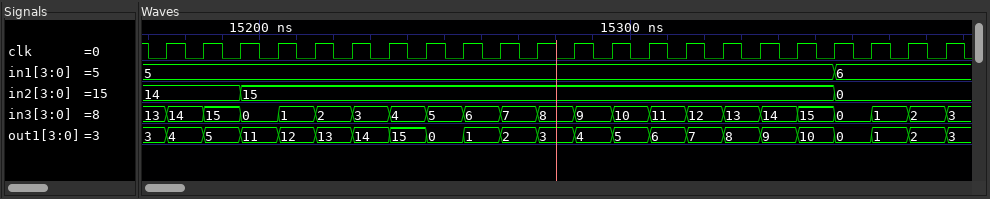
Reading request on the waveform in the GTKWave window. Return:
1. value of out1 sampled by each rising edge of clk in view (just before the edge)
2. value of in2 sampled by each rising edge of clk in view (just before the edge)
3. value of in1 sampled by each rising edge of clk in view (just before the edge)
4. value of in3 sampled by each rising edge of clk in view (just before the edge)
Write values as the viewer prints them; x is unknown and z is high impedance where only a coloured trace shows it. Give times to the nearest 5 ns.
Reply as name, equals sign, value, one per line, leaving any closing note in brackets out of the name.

value of out1 sampled by each rising edge of clk in view = 3, 4, 5, 11, 12, 13, 14, 15, 0, 1, 2, 3, 4, 5, 6, 7, 8, 9, 10, 0, 1, 2
value of in2 sampled by each rising edge of clk in view = 14, 14, 14, 15, 15, 15, 15, 15, 15, 15, 15, 15, 15, 15, 15, 15, 15, 15, 15, 0, 0, 0
value of in1 sampled by each rising edge of clk in view = 5, 5, 5, 5, 5, 5, 5, 5, 5, 5, 5, 5, 5, 5, 5, 5, 5, 5, 5, 6, 6, 6
value of in3 sampled by each rising edge of clk in view = 13, 14, 15, 0, 1, 2, 3, 4, 5, 6, 7, 8, 9, 10, 11, 12, 13, 14, 15, 0, 1, 2
